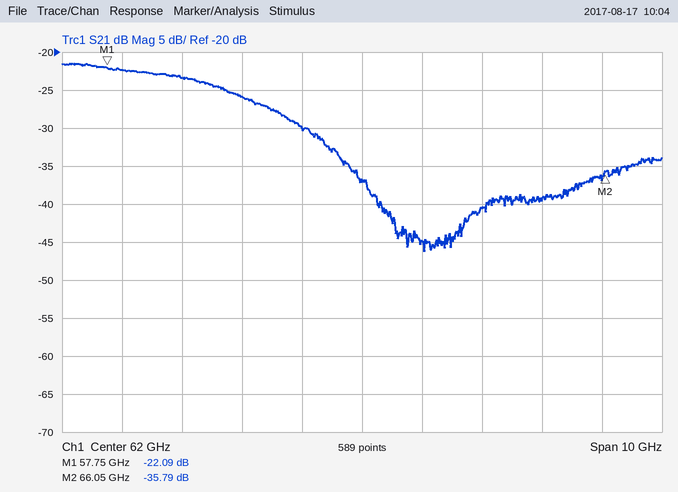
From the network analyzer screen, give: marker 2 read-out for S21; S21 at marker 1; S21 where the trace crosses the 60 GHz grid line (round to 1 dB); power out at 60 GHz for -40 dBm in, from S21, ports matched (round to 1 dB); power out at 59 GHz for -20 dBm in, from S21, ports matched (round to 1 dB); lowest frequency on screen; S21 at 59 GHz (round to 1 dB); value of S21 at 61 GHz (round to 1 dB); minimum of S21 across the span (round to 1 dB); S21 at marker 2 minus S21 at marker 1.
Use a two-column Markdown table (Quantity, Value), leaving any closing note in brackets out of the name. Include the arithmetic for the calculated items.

| Quantity | Value |
|---|---|
| marker 2 read-out for S21 | -35.79 dB |
| S21 at marker 1 | -22.09 dB |
| S21 where the trace crosses the 60 GHz grid line | -26 dB |
| power out at 60 GHz for -40 dBm in, from S21, ports matched | -40 dBm + (-26 dB) = -66 dBm |
| power out at 59 GHz for -20 dBm in, from S21, ports matched | -20 dBm + (-23 dB) = -43 dBm |
| lowest frequency on screen | 57 GHz |
| S21 at 59 GHz | -23 dB |
| value of S21 at 61 GHz | -30 dB |
| minimum of S21 across the span | -46 dB |
| S21 at marker 2 minus S21 at marker 1 | -35.79 − (-22.09) = -13.70 dB |
